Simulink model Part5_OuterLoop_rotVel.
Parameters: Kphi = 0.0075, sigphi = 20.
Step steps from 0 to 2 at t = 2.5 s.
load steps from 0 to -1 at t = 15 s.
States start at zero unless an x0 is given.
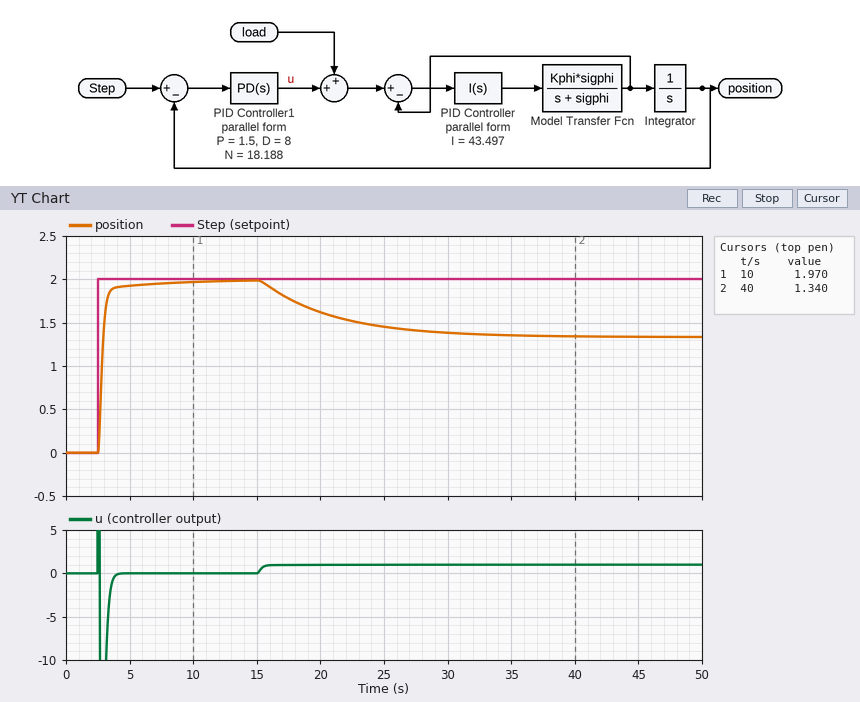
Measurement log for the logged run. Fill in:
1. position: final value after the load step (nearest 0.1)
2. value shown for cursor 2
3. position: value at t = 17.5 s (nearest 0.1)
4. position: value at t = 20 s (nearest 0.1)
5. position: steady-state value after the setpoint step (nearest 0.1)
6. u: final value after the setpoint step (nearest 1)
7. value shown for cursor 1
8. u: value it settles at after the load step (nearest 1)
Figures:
1.3
1.340
1.8
1.6
2.0
0
1.970
1
